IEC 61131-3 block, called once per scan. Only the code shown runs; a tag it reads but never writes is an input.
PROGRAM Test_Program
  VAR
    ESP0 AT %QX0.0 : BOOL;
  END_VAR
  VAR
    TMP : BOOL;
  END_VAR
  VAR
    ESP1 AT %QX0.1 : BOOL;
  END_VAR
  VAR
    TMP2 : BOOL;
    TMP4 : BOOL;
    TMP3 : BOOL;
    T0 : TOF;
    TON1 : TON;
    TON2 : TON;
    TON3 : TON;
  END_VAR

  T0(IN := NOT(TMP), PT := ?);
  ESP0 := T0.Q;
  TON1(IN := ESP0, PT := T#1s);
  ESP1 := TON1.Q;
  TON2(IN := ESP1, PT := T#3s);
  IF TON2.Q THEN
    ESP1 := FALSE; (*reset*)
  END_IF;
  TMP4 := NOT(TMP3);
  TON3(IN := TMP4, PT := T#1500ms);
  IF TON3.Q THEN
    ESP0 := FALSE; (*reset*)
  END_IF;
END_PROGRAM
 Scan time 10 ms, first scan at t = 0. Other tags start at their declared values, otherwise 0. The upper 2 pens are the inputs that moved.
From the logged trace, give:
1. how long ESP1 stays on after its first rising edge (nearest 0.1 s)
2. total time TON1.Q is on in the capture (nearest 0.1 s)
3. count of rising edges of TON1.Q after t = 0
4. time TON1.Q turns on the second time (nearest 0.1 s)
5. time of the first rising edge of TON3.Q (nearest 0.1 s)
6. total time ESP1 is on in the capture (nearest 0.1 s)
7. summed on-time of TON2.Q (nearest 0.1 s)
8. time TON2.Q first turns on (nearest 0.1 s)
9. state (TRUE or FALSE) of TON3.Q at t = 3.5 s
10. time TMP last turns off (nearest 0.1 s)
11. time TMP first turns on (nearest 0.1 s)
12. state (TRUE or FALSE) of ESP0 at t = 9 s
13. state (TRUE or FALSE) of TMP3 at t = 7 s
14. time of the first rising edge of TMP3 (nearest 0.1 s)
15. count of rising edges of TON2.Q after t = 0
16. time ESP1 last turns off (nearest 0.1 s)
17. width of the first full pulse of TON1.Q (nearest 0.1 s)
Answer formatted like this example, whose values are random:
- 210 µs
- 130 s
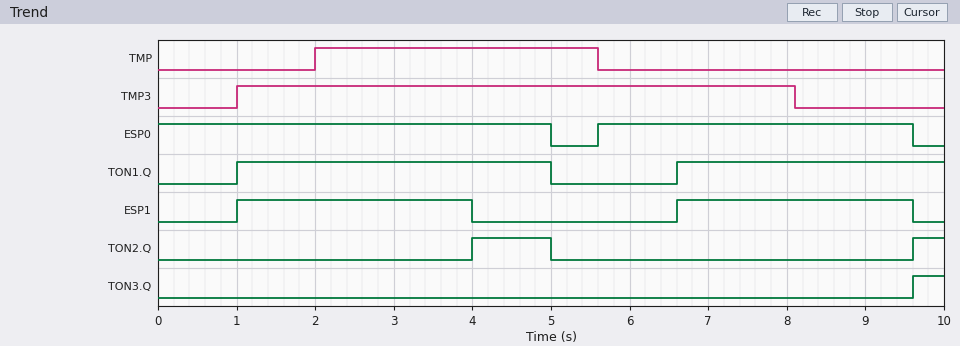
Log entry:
- 3.0 s
- 7.4 s
- 2
- 6.6 s
- 9.6 s
- 6.0 s
- 1.4 s
- 4.0 s
- FALSE
- 5.6 s
- 2.0 s
- TRUE
- TRUE
- 1.0 s
- 2
- 9.6 s
- 4.0 s
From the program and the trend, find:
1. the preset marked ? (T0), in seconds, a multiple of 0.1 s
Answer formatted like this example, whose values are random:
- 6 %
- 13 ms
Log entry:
- 3.0 s
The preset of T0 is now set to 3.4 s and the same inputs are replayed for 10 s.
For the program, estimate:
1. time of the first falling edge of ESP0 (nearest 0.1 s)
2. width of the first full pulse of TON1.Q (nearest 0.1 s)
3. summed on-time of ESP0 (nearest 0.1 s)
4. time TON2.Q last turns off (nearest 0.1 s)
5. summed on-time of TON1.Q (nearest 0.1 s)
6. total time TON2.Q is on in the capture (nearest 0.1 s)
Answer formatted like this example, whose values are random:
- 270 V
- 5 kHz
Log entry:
- 5.4 s
- 4.4 s
- 9.4 s
- 5.4 s
- 7.8 s
- 1.8 s
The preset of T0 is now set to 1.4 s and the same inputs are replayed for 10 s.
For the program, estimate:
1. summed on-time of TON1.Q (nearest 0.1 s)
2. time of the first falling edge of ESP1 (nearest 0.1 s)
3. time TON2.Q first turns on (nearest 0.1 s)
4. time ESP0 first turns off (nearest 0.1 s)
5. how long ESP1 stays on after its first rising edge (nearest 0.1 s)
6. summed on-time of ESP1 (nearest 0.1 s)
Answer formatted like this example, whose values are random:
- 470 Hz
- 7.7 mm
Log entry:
- 5.8 s
- 3.4 s
- 9.6 s
- 3.4 s
- 2.4 s
- 5.4 s
